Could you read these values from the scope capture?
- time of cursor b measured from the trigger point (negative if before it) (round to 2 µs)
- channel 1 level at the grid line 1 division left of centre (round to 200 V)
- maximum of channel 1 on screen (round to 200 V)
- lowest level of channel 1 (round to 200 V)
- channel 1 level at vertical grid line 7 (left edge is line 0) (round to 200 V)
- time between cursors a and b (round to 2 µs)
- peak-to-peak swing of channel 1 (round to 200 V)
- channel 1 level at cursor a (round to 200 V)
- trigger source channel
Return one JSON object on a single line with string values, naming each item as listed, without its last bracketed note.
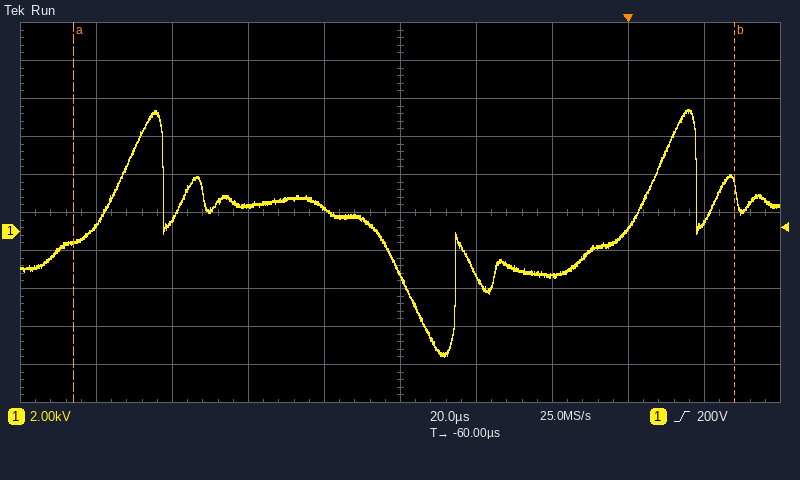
{"time of cursor b measured from the trigger point (negative if before it)": "+28 µs", "channel 1 level at the grid line 1 division left of centre": "1.2 kV", "maximum of channel 1 on screen": "6.4 kV", "lowest level of channel 1": "-6.6 kV", "channel 1 level at vertical grid line 7 (left edge is line 0)": "-2.4 kV", "time between cursors a and b": "174 µs", "peak-to-peak swing of channel 1": "13.0 kV", "channel 1 level at cursor a": "-600 V", "trigger source channel": "channel 1"}
